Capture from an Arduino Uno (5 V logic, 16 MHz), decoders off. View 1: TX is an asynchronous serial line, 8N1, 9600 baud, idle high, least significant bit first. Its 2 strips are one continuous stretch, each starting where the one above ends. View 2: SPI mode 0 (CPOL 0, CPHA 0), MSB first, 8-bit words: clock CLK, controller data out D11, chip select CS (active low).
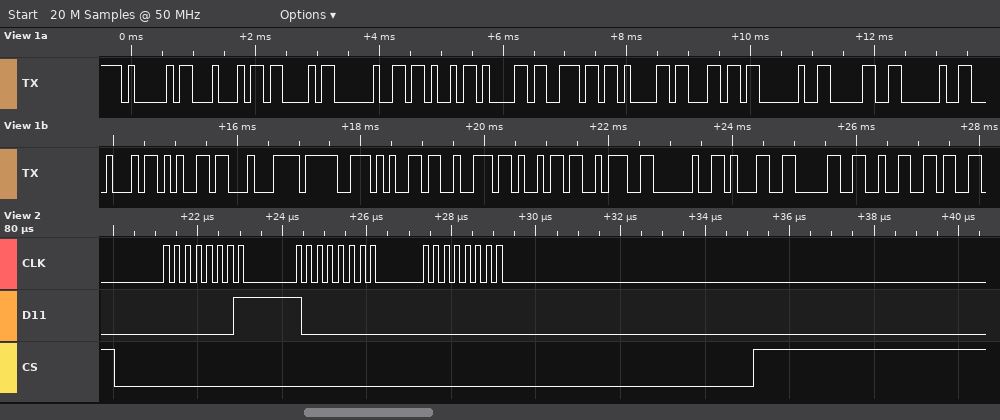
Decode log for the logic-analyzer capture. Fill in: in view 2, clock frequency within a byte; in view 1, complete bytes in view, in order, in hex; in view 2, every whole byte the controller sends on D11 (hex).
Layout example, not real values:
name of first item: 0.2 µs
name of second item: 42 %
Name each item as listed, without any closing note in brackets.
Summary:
in view 2, clock frequency within a byte: 4 MHz
in view 1, complete bytes in view, in order, in hex: 41 44 43 20 4B 61 6E 61 6C 20 30 20 44 65 C4 9F 65 72 69 3A 20 31 30 32
in view 2, every whole byte the controller sends on D11: 01 80 00
